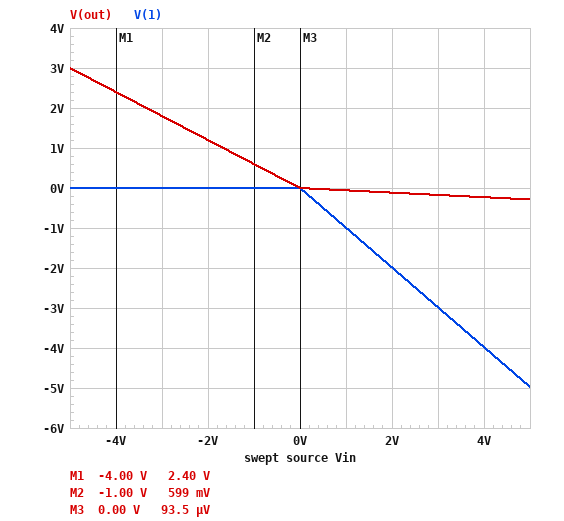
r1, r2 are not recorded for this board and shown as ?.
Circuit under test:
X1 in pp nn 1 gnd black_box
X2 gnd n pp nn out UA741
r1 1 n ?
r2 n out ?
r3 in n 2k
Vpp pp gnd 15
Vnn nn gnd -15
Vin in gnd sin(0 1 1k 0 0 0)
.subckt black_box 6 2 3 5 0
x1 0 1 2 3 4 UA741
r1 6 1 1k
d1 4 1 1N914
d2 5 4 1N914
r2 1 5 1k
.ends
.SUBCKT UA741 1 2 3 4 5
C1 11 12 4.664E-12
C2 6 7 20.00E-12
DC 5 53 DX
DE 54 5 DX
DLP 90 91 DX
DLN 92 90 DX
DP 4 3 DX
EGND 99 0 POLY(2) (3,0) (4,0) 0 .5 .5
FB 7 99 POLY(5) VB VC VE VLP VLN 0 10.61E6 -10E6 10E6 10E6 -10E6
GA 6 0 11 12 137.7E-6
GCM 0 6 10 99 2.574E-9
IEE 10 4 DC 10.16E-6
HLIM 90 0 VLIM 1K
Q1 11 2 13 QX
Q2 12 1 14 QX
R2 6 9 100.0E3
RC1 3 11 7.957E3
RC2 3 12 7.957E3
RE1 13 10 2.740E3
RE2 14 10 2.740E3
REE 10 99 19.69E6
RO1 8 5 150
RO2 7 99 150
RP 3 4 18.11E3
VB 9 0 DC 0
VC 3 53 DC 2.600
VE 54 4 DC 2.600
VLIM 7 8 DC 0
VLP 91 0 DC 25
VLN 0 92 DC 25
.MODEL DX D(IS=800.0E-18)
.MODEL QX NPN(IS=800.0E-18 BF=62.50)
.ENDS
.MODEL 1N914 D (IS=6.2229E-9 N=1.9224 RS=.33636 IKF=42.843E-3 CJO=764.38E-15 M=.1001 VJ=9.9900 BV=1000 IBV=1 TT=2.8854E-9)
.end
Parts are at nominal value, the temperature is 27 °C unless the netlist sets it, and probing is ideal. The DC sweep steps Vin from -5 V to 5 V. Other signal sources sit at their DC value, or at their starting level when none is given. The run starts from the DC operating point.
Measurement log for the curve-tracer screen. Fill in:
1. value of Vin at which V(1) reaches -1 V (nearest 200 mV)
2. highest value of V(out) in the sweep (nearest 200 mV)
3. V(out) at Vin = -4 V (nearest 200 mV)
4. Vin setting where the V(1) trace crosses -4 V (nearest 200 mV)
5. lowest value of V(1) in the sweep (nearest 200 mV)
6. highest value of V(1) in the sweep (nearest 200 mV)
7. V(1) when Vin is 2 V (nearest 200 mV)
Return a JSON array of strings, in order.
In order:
["1.0 V", "3.0 V", "2.4 V", "4.0 V", "-5.0 V", "0 V", "-2.0 V"]
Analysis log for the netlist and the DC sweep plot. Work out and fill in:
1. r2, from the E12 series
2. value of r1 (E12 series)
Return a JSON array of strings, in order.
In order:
["1.2 kΩ", "2.2 kΩ"]
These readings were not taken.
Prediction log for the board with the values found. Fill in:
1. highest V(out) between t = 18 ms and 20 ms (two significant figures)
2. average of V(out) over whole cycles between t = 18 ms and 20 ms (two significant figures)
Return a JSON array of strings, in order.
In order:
["600 mV", "170 mV"]
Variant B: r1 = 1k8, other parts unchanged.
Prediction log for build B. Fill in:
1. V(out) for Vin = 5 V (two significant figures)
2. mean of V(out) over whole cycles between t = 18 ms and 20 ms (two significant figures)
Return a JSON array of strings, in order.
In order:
["330 mV", "210 mV"]
